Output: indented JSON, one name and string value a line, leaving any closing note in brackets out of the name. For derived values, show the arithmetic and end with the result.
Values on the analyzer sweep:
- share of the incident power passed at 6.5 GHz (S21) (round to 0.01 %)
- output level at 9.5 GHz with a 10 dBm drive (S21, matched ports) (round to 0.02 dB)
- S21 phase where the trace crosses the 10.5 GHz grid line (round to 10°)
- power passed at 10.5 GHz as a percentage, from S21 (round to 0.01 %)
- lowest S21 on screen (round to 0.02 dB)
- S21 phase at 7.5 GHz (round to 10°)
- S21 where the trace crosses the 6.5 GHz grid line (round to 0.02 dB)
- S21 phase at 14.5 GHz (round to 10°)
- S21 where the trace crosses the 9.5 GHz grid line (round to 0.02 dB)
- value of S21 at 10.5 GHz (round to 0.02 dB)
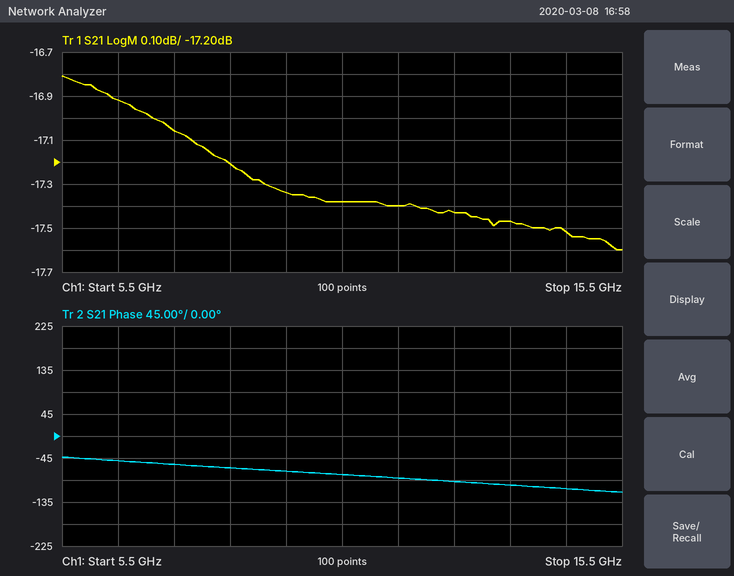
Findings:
{
  "share of the incident power passed at 6.5 GHz (S21)": "10^(-16.92/10) ≈ 2.03 %",
  "output level at 9.5 GHz with a 10 dBm drive (S21, matched ports)": "10 dBm + (-17.34 dB) = -7.34 dBm",
  "S21 phase where the trace crosses the 10.5 GHz grid line": "-80°",
  "power passed at 10.5 GHz as a percentage, from S21": "10^(-17.38/10) ≈ 1.83 %",
  "lowest S21 on screen": "-17.60 dB",
  "S21 phase at 7.5 GHz": "-60°",
  "S21 where the trace crosses the 6.5 GHz grid line": "-16.92 dB",
  "S21 phase at 14.5 GHz": "-110°",
  "S21 where the trace crosses the 9.5 GHz grid line": "-17.34 dB",
  "value of S21 at 10.5 GHz": "-17.38 dB"
}
